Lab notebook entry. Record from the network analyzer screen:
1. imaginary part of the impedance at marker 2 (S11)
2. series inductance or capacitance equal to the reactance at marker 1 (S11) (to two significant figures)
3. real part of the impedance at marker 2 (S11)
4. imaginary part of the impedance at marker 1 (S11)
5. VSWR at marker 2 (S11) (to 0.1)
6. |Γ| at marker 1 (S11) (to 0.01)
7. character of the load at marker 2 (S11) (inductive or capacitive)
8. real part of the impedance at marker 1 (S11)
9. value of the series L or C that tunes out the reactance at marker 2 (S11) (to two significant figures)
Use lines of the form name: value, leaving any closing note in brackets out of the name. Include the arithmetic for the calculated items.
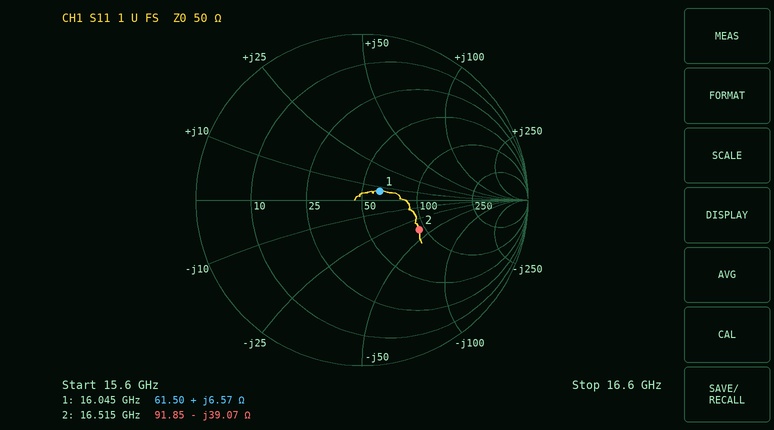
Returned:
imaginary part of the impedance at marker 2: -39.07 Ω
series inductance or capacitance equal to the reactance at marker 1 (S11): L = 6.57 Ω/(2π × 16.045 GHz) ≈ 65 pH
real part of the impedance at marker 2: 91.85 Ω
imaginary part of the impedance at marker 1: +6.57 Ω
VSWR at marker 2 (S11): 2.3
|Γ| at marker 1 (S11): 0.12
character of the load at marker 2 (S11): capacitive
real part of the impedance at marker 1: 61.50 Ω
value of the series L or C that tunes out the reactance at marker 2 (S11): L = 39.07 Ω/(2π × 16.515 GHz) ≈ 377 pH, so 380 pH to two significant figures
